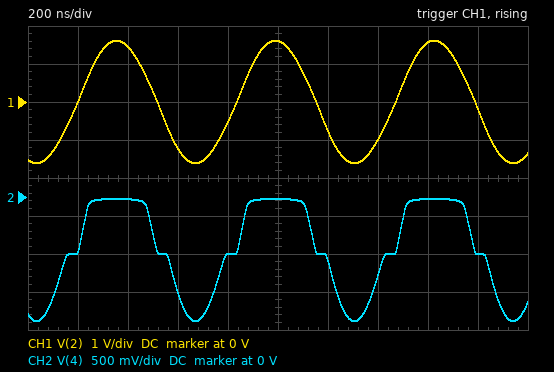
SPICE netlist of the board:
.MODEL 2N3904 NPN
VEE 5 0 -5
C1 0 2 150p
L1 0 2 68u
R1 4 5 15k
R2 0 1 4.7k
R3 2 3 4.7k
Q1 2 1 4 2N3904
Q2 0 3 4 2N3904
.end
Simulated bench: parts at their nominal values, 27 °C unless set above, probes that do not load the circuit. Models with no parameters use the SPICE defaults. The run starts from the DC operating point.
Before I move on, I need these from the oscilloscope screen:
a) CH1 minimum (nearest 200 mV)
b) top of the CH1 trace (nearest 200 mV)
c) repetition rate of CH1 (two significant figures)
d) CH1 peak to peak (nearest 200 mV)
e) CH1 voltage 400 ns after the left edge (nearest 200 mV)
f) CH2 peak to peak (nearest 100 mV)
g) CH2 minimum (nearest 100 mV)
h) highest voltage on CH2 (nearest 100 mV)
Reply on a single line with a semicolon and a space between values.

-1.6 V; 1.6 V; 1.6 MHz; 3.2 V; 1.4 V; 1.6 V; -1.6 V; 0 V
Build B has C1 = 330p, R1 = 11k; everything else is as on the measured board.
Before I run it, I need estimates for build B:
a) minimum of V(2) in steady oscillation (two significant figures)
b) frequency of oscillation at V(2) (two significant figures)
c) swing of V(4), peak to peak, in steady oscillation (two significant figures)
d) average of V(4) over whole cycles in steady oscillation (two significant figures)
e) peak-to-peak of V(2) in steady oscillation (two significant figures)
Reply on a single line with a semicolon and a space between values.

-1.8 V; 1.1 MHz; 1.8 V; -710 mV; 3.7 V
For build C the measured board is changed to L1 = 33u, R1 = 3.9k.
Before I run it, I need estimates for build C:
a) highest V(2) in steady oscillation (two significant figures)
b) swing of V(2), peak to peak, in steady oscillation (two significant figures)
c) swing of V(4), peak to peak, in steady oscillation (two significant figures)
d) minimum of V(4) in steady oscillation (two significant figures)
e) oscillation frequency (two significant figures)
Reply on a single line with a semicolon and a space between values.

3.0 V; 5.9 V; 2.9 V; -3.0 V; 2.3 MHz
